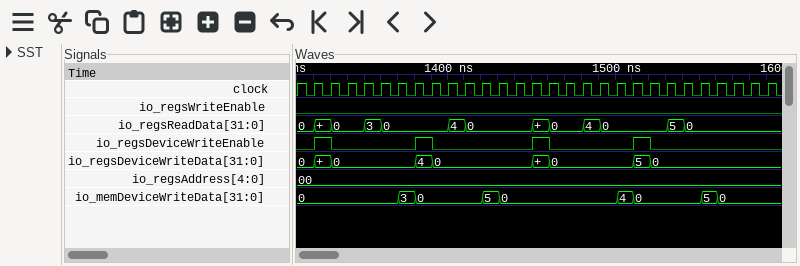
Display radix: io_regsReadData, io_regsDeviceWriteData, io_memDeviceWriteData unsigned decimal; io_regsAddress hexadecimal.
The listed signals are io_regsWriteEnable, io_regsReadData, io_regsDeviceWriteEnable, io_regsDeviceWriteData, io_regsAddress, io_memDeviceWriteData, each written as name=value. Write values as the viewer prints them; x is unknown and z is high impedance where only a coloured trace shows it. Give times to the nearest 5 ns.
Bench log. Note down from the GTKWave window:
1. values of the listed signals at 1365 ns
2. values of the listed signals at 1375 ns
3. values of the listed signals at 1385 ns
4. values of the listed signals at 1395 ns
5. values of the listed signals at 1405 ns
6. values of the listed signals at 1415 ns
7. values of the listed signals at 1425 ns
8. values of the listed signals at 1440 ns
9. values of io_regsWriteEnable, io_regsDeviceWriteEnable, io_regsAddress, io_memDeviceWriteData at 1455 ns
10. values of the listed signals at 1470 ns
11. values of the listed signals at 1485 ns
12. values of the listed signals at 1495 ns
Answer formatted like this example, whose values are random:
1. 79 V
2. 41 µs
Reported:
1. io_regsWriteEnable=0, io_regsReadData=0, io_regsDeviceWriteEnable=0, io_regsDeviceWriteData=0, io_regsAddress=00, io_memDeviceWriteData=0
2. io_regsWriteEnable=0, io_regsReadData=0, io_regsDeviceWriteEnable=0, io_regsDeviceWriteData=0, io_regsAddress=00, io_memDeviceWriteData=3
3. io_regsWriteEnable=0, io_regsReadData=0, io_regsDeviceWriteEnable=1, io_regsDeviceWriteData=4, io_regsAddress=00, io_memDeviceWriteData=0
4. io_regsWriteEnable=0, io_regsReadData=0, io_regsDeviceWriteEnable=0, io_regsDeviceWriteData=0, io_regsAddress=00, io_memDeviceWriteData=0
5. io_regsWriteEnable=0, io_regsReadData=4, io_regsDeviceWriteEnable=0, io_regsDeviceWriteData=0, io_regsAddress=00, io_memDeviceWriteData=0
6. io_regsWriteEnable=0, io_regsReadData=0, io_regsDeviceWriteEnable=0, io_regsDeviceWriteData=0, io_regsAddress=00, io_memDeviceWriteData=0
7. io_regsWriteEnable=0, io_regsReadData=0, io_regsDeviceWriteEnable=0, io_regsDeviceWriteData=0, io_regsAddress=00, io_memDeviceWriteData=5
8. io_regsWriteEnable=0, io_regsReadData=0, io_regsDeviceWriteEnable=0, io_regsDeviceWriteData=0, io_regsAddress=00, io_memDeviceWriteData=0
9. io_regsWriteEnable=0, io_regsDeviceWriteEnable=1, io_regsAddress=00, io_memDeviceWriteData=0
10. io_regsWriteEnable=0, io_regsReadData=0, io_regsDeviceWriteEnable=0, io_regsDeviceWriteData=0, io_regsAddress=00, io_memDeviceWriteData=0
11. io_regsWriteEnable=0, io_regsReadData=4, io_regsDeviceWriteEnable=0, io_regsDeviceWriteData=0, io_regsAddress=00, io_memDeviceWriteData=0
12. io_regsWriteEnable=0, io_regsReadData=0, io_regsDeviceWriteEnable=0, io_regsDeviceWriteData=0, io_regsAddress=00, io_memDeviceWriteData=0
